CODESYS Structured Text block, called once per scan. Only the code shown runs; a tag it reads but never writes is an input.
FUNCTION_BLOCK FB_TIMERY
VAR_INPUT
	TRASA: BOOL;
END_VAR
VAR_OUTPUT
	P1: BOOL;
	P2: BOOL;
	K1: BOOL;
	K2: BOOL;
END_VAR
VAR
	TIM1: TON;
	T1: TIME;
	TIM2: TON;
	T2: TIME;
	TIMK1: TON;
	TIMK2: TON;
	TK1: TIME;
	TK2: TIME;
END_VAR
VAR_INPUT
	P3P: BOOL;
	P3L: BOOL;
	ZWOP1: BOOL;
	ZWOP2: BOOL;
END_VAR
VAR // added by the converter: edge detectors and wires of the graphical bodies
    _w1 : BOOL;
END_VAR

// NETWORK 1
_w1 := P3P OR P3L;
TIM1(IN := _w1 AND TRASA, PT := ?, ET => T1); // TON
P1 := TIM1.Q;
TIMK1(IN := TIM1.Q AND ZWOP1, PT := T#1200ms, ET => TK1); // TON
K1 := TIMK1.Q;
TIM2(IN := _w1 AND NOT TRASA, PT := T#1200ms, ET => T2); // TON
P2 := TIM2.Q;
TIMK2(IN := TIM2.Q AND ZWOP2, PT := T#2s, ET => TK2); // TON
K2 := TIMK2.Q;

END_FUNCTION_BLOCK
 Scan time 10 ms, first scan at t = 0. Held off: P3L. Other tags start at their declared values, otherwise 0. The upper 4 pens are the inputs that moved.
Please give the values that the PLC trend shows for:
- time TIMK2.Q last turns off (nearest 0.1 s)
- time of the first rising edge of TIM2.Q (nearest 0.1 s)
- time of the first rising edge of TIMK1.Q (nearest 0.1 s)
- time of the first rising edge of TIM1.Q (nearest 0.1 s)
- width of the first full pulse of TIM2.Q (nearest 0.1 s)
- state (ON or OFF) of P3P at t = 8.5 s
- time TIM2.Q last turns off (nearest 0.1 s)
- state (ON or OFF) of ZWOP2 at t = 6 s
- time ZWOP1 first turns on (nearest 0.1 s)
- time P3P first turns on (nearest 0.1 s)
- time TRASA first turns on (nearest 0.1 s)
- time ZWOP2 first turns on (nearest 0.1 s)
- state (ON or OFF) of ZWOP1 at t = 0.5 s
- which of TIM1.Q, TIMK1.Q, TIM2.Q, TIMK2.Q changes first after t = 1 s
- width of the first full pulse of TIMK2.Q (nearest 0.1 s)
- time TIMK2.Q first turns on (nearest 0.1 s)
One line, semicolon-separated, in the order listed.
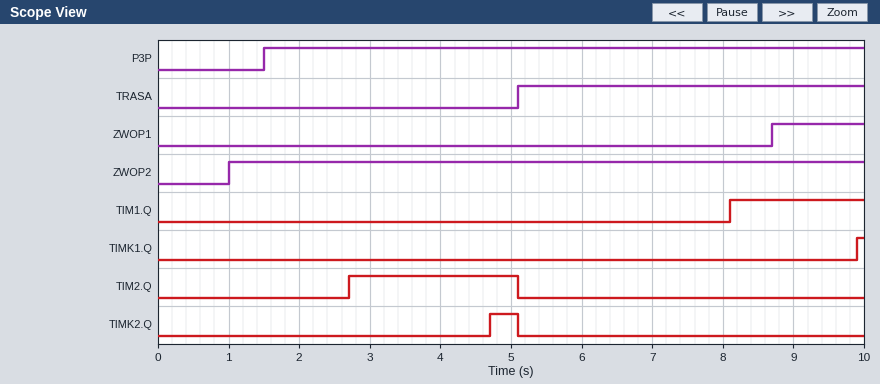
5.1 s; 2.7 s; 9.9 s; 8.1 s; 2.4 s; ON; 5.1 s; ON; 8.7 s; 1.5 s; 5.1 s; 1.0 s; OFF; TIM2.Q; 0.4 s; 4.7 s
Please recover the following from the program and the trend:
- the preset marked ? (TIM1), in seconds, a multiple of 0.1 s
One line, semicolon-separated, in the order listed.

3.0 s
